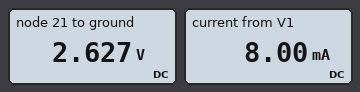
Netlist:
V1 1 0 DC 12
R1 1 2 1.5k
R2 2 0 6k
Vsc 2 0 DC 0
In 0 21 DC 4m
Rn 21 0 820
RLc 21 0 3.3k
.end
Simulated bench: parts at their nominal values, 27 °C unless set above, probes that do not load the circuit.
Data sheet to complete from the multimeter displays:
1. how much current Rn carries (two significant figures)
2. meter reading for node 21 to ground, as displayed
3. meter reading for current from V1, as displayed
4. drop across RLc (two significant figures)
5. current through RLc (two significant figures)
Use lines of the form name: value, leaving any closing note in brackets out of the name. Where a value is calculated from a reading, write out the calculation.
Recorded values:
how much current Rn carries: (2.627 V) / 820 Ω = 3.2 mA
meter reading for node 21 to ground, as displayed: 2.627 V
meter reading for current from V1, as displayed: 8.00 mA
drop across RLc: 2.627 V = 2.6 V
current through RLc: (2.627 V) / 3.3 kΩ = 800 µA
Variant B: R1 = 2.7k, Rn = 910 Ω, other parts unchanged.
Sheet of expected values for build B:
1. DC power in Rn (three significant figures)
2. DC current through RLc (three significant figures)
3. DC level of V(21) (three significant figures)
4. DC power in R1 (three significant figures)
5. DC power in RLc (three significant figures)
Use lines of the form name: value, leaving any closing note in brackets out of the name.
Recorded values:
DC power in Rn: 8.95 mW
DC current through RLc: 865 µA
DC level of V(21): 2.85 V
DC power in R1: 53.3 mW
DC power in RLc: 2.47 mW
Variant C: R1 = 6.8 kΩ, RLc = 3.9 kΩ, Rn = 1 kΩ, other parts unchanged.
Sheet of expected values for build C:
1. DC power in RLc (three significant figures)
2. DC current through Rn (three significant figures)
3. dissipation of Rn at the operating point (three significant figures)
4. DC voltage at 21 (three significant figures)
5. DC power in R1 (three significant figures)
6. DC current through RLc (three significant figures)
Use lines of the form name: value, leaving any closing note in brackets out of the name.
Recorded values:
DC power in RLc: 2.60 mW
DC current through Rn: 3.18 mA
dissipation of Rn at the operating point: 10.1 mW
DC voltage at 21: 3.18 V
DC power in R1: 21.2 mW
DC current through RLc: 816 µA
